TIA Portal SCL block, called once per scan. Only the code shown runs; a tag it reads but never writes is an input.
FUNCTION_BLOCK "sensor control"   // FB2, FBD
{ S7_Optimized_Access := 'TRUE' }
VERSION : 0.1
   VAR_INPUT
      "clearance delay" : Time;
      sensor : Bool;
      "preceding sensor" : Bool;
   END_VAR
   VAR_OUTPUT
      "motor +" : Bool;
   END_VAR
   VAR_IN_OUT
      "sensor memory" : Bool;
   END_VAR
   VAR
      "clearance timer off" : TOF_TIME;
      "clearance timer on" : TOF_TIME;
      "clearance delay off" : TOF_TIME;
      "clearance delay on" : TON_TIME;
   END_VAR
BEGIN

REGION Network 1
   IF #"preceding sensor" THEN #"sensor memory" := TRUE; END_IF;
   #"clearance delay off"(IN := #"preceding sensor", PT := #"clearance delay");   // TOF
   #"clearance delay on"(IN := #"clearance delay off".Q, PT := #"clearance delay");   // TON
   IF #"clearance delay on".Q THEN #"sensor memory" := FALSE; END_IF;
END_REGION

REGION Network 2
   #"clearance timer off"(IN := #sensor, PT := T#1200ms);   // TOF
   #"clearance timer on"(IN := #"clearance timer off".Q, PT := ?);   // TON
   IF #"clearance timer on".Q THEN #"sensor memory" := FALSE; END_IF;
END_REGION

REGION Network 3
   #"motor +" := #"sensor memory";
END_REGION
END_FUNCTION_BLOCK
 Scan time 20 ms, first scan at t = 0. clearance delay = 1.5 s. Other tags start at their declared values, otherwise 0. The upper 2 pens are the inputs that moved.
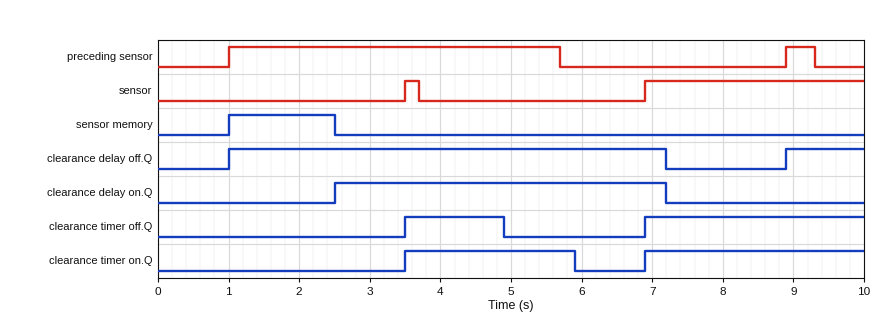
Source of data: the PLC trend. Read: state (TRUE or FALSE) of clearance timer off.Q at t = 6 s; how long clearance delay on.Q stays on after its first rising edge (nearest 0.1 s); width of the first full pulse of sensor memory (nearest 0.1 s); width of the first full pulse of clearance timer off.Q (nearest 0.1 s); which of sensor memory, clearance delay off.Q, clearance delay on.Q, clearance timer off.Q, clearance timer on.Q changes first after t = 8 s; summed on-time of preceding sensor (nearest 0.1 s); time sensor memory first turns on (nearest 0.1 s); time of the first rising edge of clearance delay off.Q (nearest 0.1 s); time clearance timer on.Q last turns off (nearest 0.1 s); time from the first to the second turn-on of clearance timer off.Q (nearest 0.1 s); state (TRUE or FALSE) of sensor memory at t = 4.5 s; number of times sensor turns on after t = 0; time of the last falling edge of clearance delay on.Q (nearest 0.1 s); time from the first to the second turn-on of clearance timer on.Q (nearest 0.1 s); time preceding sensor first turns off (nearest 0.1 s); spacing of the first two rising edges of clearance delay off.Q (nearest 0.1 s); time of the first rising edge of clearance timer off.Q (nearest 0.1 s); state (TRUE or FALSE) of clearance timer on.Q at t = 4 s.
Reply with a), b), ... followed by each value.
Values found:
a) FALSE
b) 4.7 s
c) 1.5 s
d) 1.4 s
e) clearance delay off.Q
f) 5.1 s
g) 1.0 s
h) 1.0 s
i) 5.9 s
j) 3.4 s
k) FALSE
l) 2
m) 7.2 s
n) 3.4 s
o) 5.7 s
p) 7.9 s
q) 3.5 s
r) TRUE
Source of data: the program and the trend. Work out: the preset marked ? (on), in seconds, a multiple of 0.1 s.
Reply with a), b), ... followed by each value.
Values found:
a) 1.0 s
